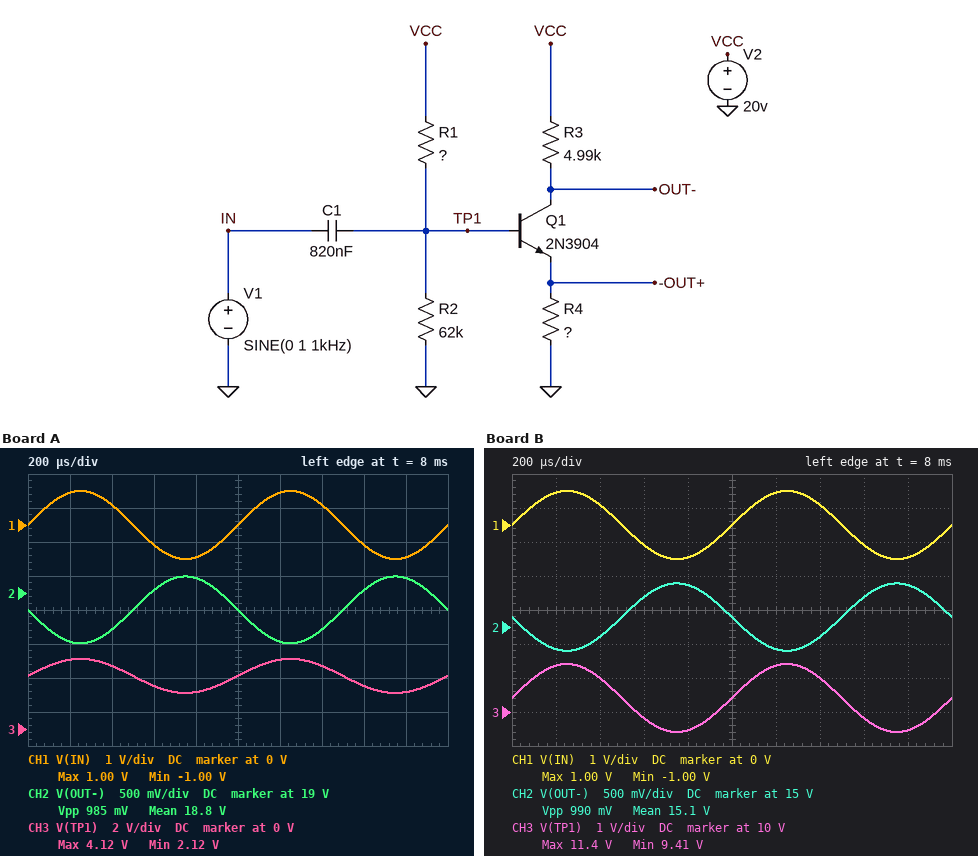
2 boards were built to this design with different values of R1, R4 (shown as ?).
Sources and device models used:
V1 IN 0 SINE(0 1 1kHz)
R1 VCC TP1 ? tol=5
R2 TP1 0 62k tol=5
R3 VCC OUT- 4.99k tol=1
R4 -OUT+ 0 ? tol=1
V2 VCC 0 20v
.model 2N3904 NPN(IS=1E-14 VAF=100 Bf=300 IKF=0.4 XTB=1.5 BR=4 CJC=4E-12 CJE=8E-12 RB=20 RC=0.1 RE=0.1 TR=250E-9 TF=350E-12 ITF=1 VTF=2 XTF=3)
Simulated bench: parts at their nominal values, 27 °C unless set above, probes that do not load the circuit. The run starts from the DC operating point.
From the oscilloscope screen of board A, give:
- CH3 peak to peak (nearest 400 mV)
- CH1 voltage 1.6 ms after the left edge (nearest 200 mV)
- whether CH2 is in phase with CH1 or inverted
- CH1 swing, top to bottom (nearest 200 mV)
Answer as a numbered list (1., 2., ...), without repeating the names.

1. 2.0 V
2. -600 mV
3. inverted
4. 2.0 V
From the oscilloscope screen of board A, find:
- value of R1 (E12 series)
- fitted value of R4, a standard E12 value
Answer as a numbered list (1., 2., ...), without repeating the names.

1. 330 kΩ
2. 10 kΩ
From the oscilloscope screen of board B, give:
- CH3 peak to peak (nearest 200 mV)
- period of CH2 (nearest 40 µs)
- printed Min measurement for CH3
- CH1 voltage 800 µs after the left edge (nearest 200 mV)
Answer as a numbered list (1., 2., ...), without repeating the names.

1. 2.0 V
2. 1.00 ms
3. 9.41 V
4. -1.0 V
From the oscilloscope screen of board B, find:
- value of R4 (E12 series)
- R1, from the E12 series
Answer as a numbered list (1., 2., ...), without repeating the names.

1. 10 kΩ
2. 56 kΩ
